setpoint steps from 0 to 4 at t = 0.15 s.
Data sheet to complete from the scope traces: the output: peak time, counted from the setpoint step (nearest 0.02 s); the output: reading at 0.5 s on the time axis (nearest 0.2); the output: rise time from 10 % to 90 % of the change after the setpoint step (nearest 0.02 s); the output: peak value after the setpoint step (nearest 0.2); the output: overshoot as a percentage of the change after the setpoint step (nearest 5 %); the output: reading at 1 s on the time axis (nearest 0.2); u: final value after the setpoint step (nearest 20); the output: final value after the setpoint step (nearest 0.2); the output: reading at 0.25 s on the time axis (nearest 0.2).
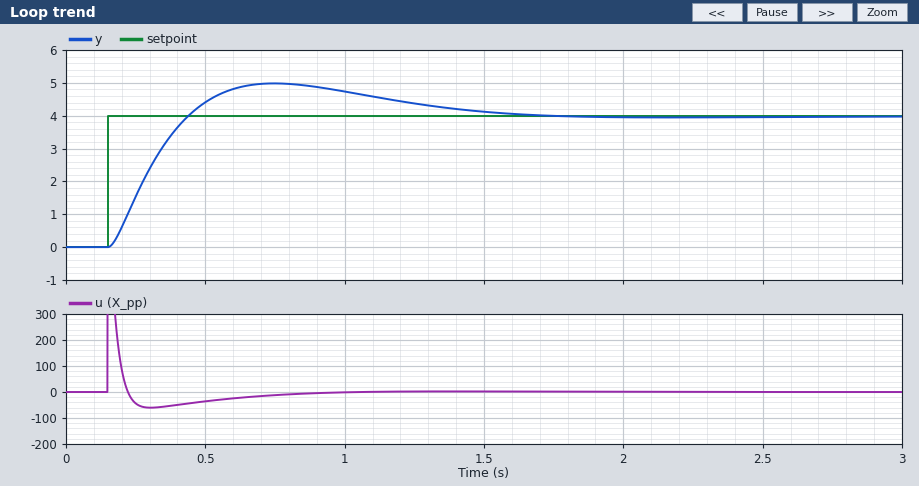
0.60 s
4.4
0.20 s
5.0
25 %
4.8
0
4.0
1.6
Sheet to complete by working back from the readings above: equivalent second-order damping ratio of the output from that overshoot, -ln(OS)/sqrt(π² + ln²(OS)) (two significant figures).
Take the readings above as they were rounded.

0.40
